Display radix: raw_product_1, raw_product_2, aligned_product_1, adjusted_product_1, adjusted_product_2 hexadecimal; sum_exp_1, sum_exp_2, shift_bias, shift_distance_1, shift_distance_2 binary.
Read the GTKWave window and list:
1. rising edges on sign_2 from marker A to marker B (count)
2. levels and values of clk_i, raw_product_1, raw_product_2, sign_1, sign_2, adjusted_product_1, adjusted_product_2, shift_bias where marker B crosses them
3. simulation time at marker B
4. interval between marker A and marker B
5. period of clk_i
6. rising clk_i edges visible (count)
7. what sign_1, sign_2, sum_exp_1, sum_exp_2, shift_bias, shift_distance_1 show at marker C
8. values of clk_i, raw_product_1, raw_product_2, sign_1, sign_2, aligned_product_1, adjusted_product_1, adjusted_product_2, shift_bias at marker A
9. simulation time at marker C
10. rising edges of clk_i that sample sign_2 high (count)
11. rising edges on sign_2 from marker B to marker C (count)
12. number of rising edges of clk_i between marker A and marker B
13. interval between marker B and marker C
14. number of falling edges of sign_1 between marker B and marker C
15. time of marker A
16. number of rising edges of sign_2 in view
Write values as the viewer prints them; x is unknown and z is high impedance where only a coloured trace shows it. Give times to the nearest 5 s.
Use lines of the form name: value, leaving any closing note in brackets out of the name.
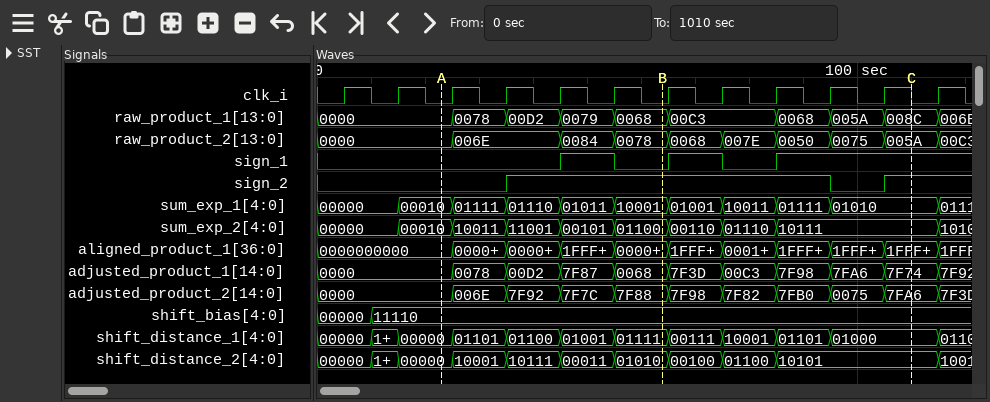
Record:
rising edges on sign_2 from marker A to marker B: 1
levels and values of clk_i, raw_product_1, raw_product_2, sign_1, sign_2, adjusted_product_1, adjusted_product_2, shift_bias where marker B crosses them: clk_i=0, raw_product_1=0068, raw_product_2=0078, sign_1=0, sign_2=1, adjusted_product_1=0068, adjusted_product_2=7F88, shift_bias=11110
simulation time at marker B: 65 s
interval between marker A and marker B: 40 s
period of clk_i: 10 s
rising clk_i edges visible: 12
what sign_1, sign_2, sum_exp_1, sum_exp_2, shift_bias, shift_distance_1 show at marker C: sign_1=1, sign_2=1, sum_exp_1=01010, sum_exp_2=10111, shift_bias=11110, shift_distance_1=01000
values of clk_i, raw_product_1, raw_product_2, sign_1, sign_2, aligned_product_1, adjusted_product_1, adjusted_product_2, shift_bias at marker A: clk_i=0, raw_product_1=0000, raw_product_2=0000, sign_1=0, sign_2=0, aligned_product_1=0000000000, adjusted_product_1=0000, adjusted_product_2=0000, shift_bias=11110
simulation time at marker C: 110 s
rising edges of clk_i that sample sign_2 high: 7
rising edges on sign_2 from marker B to marker C: 1
number of rising edges of clk_i between marker A and marker B: 4
interval between marker B and marker C: 45 s
number of falling edges of sign_1 between marker B and marker C: 1
time of marker A: 25 s
number of rising edges of sign_2 in view: 2
